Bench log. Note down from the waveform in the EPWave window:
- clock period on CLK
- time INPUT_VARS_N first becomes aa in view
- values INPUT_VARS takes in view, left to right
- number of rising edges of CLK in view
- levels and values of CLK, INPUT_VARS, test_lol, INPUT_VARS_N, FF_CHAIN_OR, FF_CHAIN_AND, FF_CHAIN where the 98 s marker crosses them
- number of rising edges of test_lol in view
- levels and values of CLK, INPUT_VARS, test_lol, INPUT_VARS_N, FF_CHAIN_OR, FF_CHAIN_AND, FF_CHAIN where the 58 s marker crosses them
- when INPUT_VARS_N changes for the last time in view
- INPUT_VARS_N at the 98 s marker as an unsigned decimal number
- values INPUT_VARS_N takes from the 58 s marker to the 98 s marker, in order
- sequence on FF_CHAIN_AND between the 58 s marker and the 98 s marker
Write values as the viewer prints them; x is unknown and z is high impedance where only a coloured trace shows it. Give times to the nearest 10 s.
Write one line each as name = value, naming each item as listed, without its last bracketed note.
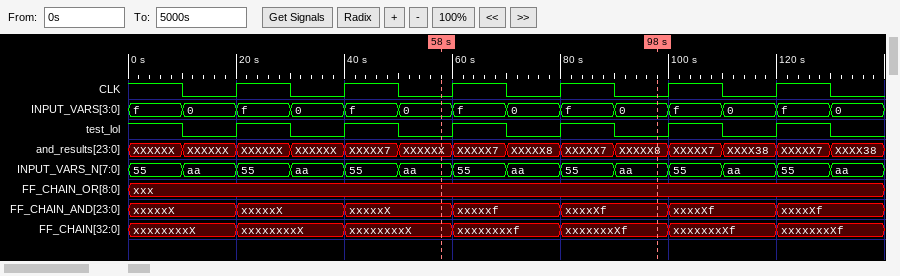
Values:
clock period on CLK = 20 s
time INPUT_VARS_N first becomes aa in view = 10 s
values INPUT_VARS takes in view, left to right = f, 0, f, 0, f, 0, f, 0, f, 0, f, 0, f, 0
number of rising edges of CLK in view = 6
levels and values of CLK, INPUT_VARS, test_lol, INPUT_VARS_N, FF_CHAIN_OR, FF_CHAIN_AND, FF_CHAIN where the 98 s marker crosses them = CLK=0, INPUT_VARS=0, test_lol=0, INPUT_VARS_N=aa, FF_CHAIN_OR=xxx, FF_CHAIN_AND=xxxxXf, FF_CHAIN=xxxxxxxXf
number of rising edges of test_lol in view = 6
levels and values of CLK, INPUT_VARS, test_lol, INPUT_VARS_N, FF_CHAIN_OR, FF_CHAIN_AND, FF_CHAIN where the 58 s marker crosses them = CLK=0, INPUT_VARS=0, test_lol=0, INPUT_VARS_N=aa, FF_CHAIN_OR=xxx, FF_CHAIN_AND=xxxxxX, FF_CHAIN=xxxxxxxxX
when INPUT_VARS_N changes for the last time in view = 130 s
INPUT_VARS_N at the 98 s marker as an unsigned decimal number = 170
values INPUT_VARS_N takes from the 58 s marker to the 98 s marker, in order = aa, 55, aa, 55, aa
sequence on FF_CHAIN_AND between the 58 s marker and the 98 s marker = xxxxxX, xxxxxf, xxxxXf
